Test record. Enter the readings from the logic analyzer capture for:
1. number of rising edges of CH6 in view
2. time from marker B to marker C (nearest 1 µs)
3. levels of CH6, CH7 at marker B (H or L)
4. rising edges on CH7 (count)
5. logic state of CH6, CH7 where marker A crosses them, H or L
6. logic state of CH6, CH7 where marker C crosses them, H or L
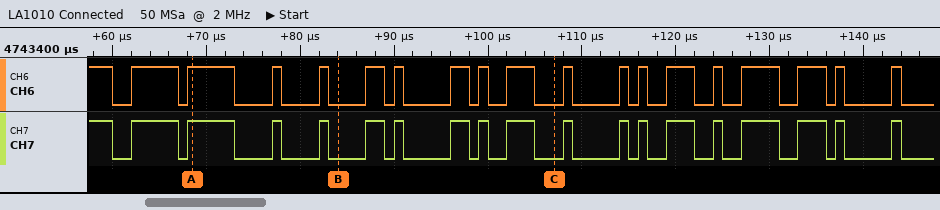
18
23 µs
CH6=L, CH7=L
18
CH6=H, CH7=H
CH6=L, CH7=L
